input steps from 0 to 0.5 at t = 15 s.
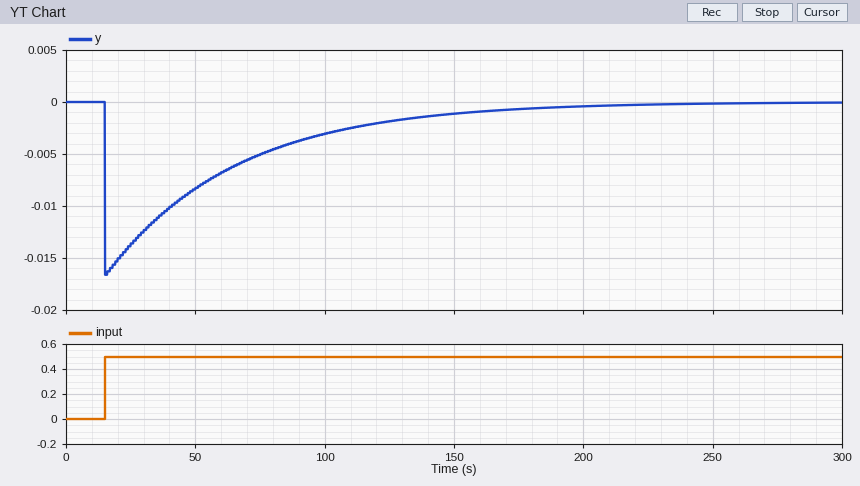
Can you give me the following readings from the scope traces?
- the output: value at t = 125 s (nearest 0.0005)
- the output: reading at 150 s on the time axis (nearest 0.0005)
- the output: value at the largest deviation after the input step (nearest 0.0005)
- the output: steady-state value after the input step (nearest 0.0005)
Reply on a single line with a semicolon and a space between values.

-0.0020; -0.0010; -0.0165; 0.0000
